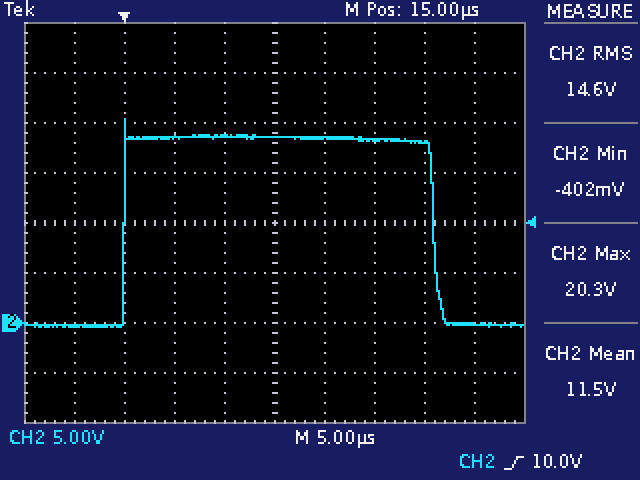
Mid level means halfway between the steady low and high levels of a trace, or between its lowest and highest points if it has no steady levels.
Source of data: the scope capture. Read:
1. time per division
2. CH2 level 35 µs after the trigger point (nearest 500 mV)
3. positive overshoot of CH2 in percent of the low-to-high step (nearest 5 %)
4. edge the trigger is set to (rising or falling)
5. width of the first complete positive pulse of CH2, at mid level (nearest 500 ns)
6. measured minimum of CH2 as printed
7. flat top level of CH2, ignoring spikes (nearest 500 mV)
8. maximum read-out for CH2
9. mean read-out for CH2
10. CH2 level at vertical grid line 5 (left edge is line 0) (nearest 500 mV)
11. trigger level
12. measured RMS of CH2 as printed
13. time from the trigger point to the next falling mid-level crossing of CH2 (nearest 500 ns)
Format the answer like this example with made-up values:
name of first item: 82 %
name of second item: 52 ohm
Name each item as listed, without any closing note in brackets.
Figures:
time per division: 5 µs
CH2 level 35 µs after the trigger point: 0.0 V
positive overshoot of CH2 in percent of the low-to-high step: 10 %
edge the trigger is set to: rising
width of the first complete positive pulse of CH2, at mid level: 31.0 µs
measured minimum of CH2 as printed: -402 mV
flat top level of CH2, ignoring spikes: 18.5 V
maximum read-out for CH2: 20.3 V
mean read-out for CH2: 11.5 V
CH2 level at vertical grid line 5 (left edge is line 0): 18.5 V
trigger level: 10.0 V
measured RMS of CH2 as printed: 14.6 V
time from the trigger point to the next falling mid-level crossing of CH2: 31.0 µs
